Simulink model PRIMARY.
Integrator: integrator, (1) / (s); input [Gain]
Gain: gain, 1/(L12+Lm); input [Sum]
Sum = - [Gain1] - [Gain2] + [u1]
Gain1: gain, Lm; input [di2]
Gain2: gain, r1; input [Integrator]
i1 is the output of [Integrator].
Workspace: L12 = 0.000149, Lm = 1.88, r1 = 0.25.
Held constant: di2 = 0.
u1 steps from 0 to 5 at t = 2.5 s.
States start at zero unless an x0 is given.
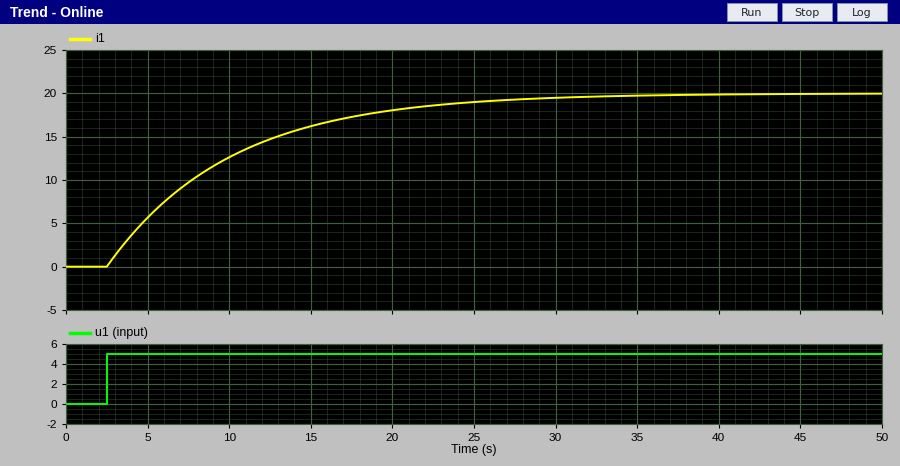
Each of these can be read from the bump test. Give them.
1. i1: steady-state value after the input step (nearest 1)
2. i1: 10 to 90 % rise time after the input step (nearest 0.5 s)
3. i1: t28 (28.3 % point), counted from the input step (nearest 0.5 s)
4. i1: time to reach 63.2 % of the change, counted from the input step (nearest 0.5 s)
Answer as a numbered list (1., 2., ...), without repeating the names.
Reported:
1. 20
2. 16.5 s
3. 2.5 s
4. 7.5 s
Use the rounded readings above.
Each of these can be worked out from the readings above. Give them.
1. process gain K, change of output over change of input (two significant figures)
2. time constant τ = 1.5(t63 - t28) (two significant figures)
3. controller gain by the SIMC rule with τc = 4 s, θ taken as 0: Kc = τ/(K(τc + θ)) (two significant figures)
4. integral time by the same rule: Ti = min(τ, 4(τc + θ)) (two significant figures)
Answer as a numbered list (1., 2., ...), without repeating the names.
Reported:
1. 4.0
2. 7.5 s
3. 0.47
4. 7.5 s
